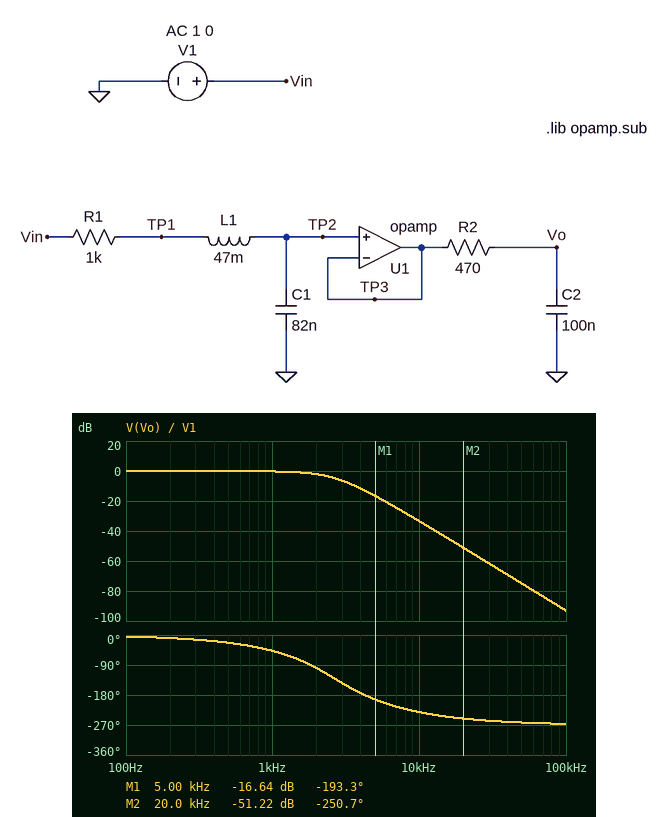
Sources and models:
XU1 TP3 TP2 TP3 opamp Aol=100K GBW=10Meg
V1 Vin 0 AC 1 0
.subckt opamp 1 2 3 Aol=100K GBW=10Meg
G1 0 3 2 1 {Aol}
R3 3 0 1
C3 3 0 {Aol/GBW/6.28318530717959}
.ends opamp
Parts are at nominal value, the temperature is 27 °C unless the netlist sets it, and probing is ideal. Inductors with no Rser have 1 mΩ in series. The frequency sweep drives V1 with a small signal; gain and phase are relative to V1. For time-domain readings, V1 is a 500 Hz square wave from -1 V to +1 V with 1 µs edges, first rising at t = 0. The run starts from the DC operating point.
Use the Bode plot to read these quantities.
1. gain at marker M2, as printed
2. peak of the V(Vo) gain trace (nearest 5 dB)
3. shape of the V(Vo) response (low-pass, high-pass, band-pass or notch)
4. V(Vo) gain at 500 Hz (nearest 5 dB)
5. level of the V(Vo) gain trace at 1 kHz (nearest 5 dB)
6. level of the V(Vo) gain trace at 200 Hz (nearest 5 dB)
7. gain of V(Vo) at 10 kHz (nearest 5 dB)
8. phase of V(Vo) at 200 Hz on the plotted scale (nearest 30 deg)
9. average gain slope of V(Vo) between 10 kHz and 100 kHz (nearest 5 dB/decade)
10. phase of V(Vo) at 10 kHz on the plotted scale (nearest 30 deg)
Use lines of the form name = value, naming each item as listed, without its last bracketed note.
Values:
gain at marker M2, as printed = -51.22 dB
peak of the V(Vo) gain trace = 0 dB
shape of the V(Vo) response = low-pass
V(Vo) gain at 500 Hz = 0 dB
level of the V(Vo) gain trace at 1 kHz = 0 dB
level of the V(Vo) gain trace at 200 Hz = 0 dB
gain of V(Vo) at 10 kHz = -35 dB
phase of V(Vo) at 200 Hz on the plotted scale = 0 deg
average gain slope of V(Vo) between 10 kHz and 100 kHz = -60 dB/decade
phase of V(Vo) at 10 kHz on the plotted scale = -240 deg
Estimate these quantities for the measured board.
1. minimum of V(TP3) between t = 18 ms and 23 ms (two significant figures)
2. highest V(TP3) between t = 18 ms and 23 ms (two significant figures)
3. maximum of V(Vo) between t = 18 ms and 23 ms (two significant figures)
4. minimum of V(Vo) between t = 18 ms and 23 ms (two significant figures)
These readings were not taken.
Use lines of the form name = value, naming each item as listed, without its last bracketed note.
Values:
minimum of V(TP3) between t = 18 ms and 23 ms = -1.1 V
highest V(TP3) between t = 18 ms and 23 ms = 1.1 V
maximum of V(Vo) between t = 18 ms and 23 ms = 1.1 V
minimum of V(Vo) between t = 18 ms and 23 ms = -1.1 V
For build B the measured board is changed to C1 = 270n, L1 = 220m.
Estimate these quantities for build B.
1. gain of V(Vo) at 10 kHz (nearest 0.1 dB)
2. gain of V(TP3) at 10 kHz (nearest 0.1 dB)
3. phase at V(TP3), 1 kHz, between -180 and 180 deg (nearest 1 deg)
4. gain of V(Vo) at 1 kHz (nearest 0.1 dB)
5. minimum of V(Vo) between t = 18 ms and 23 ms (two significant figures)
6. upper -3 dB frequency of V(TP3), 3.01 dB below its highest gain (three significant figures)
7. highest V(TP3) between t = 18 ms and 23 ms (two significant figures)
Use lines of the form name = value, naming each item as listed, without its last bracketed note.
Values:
gain of V(Vo) at 10 kHz = -57.3 dB
gain of V(TP3) at 10 kHz = -47.4 dB
phase at V(TP3), 1 kHz, between -180 and 180 deg = -128 deg
gain of V(Vo) at 1 kHz = -7.1 dB
minimum of V(Vo) between t = 18 ms and 23 ms = -1.3 V
upper -3 dB frequency of V(TP3), 3.01 dB below its highest gain = 747 Hz
highest V(TP3) between t = 18 ms and 23 ms = 1.3 V
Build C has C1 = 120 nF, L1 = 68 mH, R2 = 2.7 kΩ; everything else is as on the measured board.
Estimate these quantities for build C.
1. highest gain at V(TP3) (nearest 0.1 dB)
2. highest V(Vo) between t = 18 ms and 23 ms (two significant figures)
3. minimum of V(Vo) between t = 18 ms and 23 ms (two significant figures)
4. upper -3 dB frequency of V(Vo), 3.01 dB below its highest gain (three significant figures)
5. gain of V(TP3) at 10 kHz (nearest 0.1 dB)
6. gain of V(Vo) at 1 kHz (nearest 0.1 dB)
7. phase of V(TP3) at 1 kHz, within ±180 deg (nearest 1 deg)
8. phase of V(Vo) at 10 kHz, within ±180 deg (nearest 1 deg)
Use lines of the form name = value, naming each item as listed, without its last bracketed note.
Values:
highest gain at V(TP3) = 0.1 dB
highest V(Vo) between t = 18 ms and 23 ms = 930 mV
minimum of V(Vo) between t = 18 ms and 23 ms = -930 mV
upper -3 dB frequency of V(Vo), 3.01 dB below its highest gain = 598 Hz
gain of V(TP3) at 10 kHz = -30.1 dB
gain of V(Vo) at 1 kHz = -6.0 dB
phase of V(TP3) at 1 kHz, within ±180 deg = -48 deg
phase of V(Vo) at 10 kHz, within ±180 deg = 107 deg
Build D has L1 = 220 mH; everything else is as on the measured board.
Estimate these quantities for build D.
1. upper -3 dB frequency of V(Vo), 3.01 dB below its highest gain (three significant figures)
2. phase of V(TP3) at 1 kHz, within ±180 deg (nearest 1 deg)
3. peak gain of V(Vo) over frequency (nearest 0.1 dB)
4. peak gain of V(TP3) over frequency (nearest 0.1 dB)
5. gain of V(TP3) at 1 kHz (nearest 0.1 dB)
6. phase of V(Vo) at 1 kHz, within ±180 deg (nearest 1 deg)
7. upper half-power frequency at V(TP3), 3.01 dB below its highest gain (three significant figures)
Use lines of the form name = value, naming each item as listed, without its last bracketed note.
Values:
upper -3 dB frequency of V(Vo), 3.01 dB below its highest gain = 1.38 kHz
phase of V(TP3) at 1 kHz, within ±180 deg = -61 deg
peak gain of V(Vo) over frequency = 4.3 dB
peak gain of V(TP3) over frequency = 4.7 dB
gain of V(TP3) at 1 kHz = 4.6 dB
phase of V(Vo) at 1 kHz, within ±180 deg = -77 deg
upper half-power frequency at V(TP3), 3.01 dB below its highest gain = 1.40 kHz
